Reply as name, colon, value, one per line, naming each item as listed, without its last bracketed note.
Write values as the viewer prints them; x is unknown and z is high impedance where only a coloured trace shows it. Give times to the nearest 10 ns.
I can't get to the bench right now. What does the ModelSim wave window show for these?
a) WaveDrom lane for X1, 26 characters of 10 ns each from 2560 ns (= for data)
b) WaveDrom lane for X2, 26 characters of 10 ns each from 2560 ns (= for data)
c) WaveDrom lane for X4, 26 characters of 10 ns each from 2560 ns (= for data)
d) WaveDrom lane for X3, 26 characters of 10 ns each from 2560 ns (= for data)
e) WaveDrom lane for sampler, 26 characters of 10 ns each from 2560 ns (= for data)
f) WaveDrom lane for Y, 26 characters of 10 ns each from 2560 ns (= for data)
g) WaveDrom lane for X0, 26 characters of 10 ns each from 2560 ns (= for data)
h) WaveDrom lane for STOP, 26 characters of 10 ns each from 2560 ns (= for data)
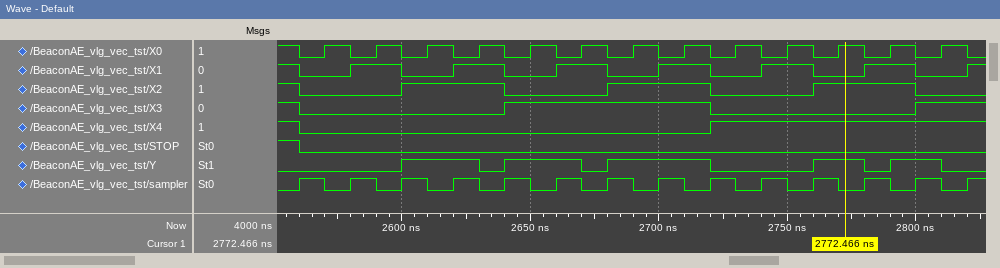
WaveDrom lane for X1, 26 characters of 10 ns each from 2560 ns: {name: 'X1', wave: '0.1.0.1.0.1.0.1.0.1.0.1.0.'}
WaveDrom lane for X2, 26 characters of 10 ns each from 2560 ns: {name: 'X2', wave: '0...1...0...1...0...1...0.'}
WaveDrom lane for X4, 26 characters of 10 ns each from 2560 ns: {name: 'X4', wave: '0...............1.........'}
WaveDrom lane for X3, 26 characters of 10 ns each from 2560 ns: {name: 'X3', wave: '0.......1.......0.......1.'}
WaveDrom lane for sampler, 26 characters of 10 ns each from 2560 ns: {name: 'sampler', wave: '10101010101010101010101010'}
WaveDrom lane for Y, 26 characters of 10 ns each from 2560 ns: {name: 'Y', wave: '0...1..01..01...0...1.01.0'}
WaveDrom lane for X0, 26 characters of 10 ns each from 2560 ns: {name: 'X0', wave: '01010101010101010101010101'}
WaveDrom lane for STOP, 26 characters of 10 ns each from 2560 ns: {name: 'STOP', wave: '0.........................'}
